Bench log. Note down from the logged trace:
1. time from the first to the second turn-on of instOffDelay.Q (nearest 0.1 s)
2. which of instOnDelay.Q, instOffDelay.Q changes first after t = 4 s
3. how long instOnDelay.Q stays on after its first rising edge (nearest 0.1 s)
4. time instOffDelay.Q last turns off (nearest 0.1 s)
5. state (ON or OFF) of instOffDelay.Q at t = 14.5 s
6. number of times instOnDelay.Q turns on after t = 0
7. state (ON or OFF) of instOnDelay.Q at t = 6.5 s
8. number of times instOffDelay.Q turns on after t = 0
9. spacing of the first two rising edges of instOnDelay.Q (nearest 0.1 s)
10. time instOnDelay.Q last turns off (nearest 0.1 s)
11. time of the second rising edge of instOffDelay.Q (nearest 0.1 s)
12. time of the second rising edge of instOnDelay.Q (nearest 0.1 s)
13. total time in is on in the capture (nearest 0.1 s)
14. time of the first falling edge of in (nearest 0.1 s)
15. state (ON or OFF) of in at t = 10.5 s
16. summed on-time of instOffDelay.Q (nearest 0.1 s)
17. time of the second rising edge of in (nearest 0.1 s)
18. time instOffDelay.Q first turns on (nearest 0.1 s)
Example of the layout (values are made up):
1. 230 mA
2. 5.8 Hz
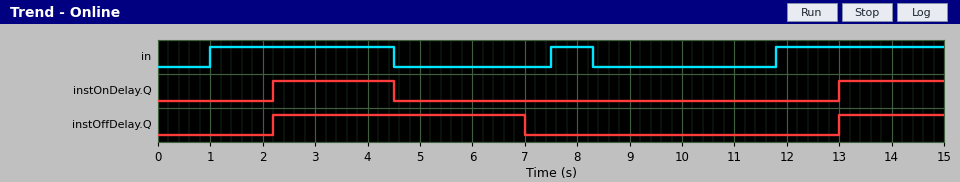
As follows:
1. 10.8 s
2. instOnDelay.Q
3. 2.3 s
4. 7.0 s
5. ON
6. 2
7. OFF
8. 2
9. 10.8 s
10. 4.5 s
11. 13.0 s
12. 13.0 s
13. 7.5 s
14. 4.5 s
15. OFF
16. 6.8 s
17. 7.5 s
18. 2.2 s
